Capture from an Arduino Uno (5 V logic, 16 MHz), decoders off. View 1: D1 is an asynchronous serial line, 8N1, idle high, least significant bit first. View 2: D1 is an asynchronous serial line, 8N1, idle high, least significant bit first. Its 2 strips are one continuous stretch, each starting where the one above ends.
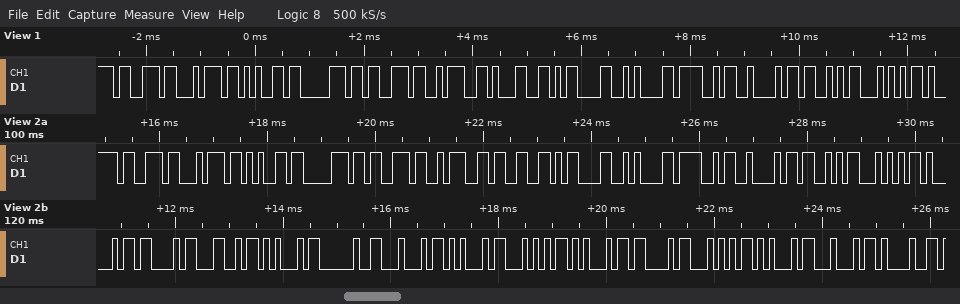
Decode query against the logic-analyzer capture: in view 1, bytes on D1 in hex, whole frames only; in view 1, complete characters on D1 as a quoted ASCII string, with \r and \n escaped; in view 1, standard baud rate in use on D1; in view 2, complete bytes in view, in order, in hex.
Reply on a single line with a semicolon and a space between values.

0x73 0x74 0x65 0x70 0x73 0x3A 0x31 0x0D 0x0A 0x4F 0x42 0x53 0x54; "steps:1\r\nOBST"; 9600 baud; 73 74 65 70 73 3A 33 0D 0A 4F 42 53 54 41 43 4C 45 20 44 45 54 45 43 54 45 44 21
